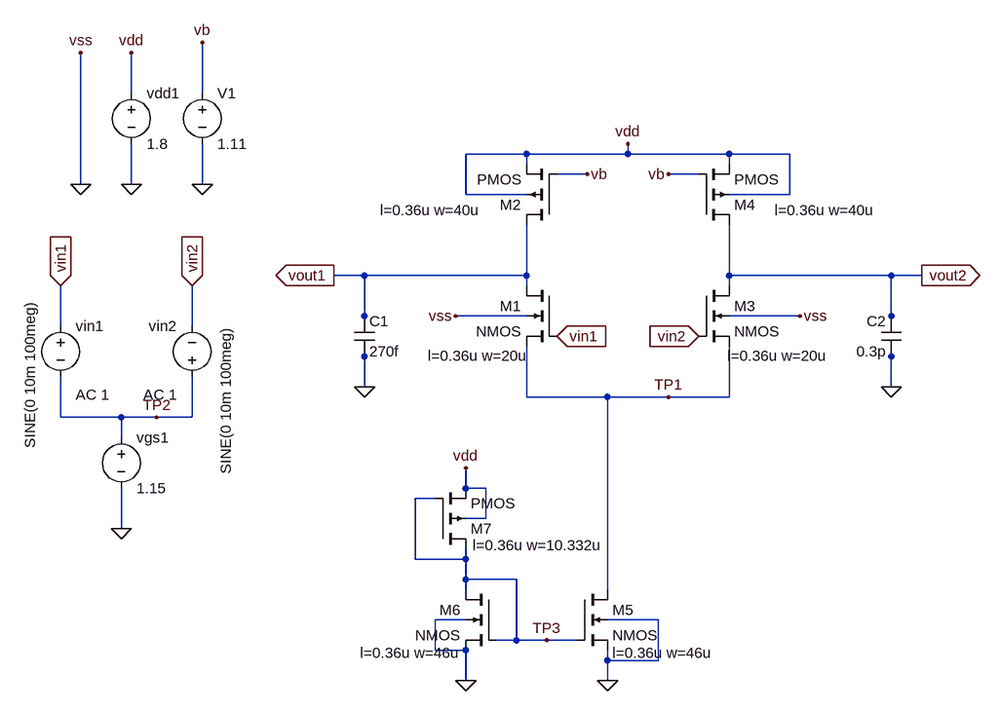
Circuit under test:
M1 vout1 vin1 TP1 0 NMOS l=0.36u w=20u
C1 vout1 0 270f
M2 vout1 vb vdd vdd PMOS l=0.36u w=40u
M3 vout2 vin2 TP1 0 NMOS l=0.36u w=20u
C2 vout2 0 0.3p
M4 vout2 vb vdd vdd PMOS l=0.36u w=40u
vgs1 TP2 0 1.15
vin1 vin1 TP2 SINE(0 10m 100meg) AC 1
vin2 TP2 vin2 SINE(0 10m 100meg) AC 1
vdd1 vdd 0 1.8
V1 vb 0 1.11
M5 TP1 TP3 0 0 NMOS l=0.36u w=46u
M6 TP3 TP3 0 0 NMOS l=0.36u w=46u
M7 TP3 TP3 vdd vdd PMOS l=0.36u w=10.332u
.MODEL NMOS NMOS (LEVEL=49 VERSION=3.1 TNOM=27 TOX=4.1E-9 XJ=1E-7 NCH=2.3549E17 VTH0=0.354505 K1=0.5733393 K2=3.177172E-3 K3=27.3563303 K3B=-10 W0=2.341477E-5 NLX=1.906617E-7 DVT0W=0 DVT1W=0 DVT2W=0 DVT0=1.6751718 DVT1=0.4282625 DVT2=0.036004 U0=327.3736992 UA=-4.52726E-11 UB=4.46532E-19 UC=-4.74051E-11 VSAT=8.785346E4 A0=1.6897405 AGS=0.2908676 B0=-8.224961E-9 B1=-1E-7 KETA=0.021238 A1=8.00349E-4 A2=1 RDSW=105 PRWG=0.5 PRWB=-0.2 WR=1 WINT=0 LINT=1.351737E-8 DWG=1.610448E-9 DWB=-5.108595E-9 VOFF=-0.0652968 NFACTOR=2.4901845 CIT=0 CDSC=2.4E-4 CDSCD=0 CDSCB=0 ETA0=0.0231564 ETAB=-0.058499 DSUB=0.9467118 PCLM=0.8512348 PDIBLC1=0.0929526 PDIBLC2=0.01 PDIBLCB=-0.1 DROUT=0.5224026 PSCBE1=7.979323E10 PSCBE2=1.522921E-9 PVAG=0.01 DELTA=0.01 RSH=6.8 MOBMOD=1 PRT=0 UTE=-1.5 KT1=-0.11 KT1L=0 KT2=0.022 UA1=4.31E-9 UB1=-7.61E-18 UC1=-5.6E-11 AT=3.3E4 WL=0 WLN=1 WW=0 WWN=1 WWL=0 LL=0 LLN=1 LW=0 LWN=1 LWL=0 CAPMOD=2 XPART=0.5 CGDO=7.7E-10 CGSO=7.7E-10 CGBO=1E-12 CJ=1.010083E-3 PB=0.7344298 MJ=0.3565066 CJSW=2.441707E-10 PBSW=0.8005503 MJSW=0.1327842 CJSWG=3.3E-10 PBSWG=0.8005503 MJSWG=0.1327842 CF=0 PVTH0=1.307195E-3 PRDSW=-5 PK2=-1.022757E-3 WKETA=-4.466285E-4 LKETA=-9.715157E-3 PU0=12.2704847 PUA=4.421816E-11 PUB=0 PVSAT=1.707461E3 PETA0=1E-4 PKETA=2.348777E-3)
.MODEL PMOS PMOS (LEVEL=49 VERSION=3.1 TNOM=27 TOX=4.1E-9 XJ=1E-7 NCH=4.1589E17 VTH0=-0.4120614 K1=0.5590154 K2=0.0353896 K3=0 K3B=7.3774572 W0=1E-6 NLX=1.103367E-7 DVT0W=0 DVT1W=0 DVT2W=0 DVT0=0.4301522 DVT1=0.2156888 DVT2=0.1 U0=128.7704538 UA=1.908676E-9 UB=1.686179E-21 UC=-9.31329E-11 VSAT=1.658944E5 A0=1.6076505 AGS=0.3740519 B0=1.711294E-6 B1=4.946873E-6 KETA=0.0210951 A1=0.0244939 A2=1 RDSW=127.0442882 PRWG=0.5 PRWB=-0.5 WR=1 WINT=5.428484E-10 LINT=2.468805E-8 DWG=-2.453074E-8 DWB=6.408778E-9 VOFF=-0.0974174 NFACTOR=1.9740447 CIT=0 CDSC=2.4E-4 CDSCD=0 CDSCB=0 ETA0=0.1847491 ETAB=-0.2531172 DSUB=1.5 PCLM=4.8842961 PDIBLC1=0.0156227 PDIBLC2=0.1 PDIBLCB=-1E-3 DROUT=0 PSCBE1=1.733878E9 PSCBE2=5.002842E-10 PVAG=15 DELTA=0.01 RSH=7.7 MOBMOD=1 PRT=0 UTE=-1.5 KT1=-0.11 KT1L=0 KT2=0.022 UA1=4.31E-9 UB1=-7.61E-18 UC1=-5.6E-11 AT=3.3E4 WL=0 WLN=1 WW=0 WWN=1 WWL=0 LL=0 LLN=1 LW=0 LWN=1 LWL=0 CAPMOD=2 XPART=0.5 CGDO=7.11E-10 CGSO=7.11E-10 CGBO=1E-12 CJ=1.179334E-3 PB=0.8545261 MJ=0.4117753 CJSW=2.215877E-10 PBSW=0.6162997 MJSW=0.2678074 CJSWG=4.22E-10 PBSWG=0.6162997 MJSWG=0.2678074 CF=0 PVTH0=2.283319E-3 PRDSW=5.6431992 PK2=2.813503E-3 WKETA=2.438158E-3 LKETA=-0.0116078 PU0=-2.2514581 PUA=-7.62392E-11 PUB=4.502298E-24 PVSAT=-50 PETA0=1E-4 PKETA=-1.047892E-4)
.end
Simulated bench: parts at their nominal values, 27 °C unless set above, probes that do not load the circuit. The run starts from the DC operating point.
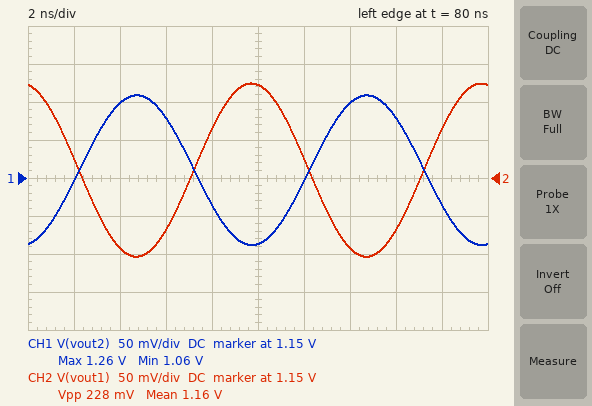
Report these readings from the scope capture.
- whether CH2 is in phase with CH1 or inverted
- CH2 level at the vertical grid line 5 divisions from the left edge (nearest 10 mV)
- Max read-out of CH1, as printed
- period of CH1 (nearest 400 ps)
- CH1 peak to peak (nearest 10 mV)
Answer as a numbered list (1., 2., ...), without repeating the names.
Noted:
1. inverted
2. 1.27 V
3. 1.26 V
4. 10.0 ns
5. 200 mV
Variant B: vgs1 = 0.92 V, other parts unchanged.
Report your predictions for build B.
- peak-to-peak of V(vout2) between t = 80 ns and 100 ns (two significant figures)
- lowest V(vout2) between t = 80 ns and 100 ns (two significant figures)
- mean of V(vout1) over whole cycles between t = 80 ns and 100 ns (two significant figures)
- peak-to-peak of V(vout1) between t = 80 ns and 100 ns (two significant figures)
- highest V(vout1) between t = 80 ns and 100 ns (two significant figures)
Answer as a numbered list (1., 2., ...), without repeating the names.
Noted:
1. 190 mV
2. 1.4 V
3. 1.5 V
4. 220 mV
5. 1.6 V
